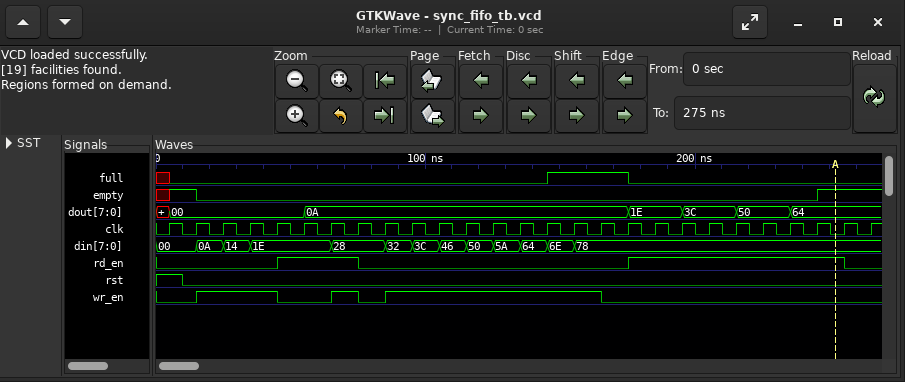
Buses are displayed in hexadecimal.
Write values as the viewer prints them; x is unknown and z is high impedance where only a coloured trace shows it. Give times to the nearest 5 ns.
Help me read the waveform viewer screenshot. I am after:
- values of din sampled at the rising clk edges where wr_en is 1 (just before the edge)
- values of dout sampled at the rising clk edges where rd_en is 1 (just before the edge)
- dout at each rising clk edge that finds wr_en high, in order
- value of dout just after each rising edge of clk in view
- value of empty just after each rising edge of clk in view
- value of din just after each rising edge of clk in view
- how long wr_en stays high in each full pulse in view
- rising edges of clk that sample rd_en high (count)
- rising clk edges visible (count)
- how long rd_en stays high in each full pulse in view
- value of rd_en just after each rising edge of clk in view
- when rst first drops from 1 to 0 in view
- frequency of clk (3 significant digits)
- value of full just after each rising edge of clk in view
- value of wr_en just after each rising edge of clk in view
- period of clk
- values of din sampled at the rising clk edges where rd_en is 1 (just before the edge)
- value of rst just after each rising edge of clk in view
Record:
0A, 14, 1E, 28, 32, 3C, 46, 50, 5A, 64, 6E, 78
00, 0A, 0A, 1E, 1E, 3C, 3C, 50, 50, 64, 64
00, 00, 00, 0A, 0A, 0A, 0A, 0A, 0A, 0A, 0A, 0A
00, 00, 00, 00, 00, 0A, 0A, 0A, 0A, 0A, 0A, 0A, 0A, 0A, 0A, 0A, 0A, 1E, 1E, 3C, 3C, 50, 50, 64, 64, 64, 64
1 0 0 0 0 0 0 0 0 0 0 0 0 0 0 0 0 0 0 0 0 0 0 0 1 1 1
00, 0A, 14, 1E, 1E, 1E, 28, 28, 32, 3C, 46, 50, 5A, 64, 6E, 78, 78, 78, 78, 78, 78, 78, 78, 78, 78, 78, 78
30 ns, 10 ns, 80 ns
11
27
30 ns, 80 ns
0 0 0 0 1 1 1 0 0 0 0 0 0 0 0 0 0 1 1 1 1 1 1 1 1 0 0
10 ns
100 MHz
0 0 0 0 0 0 0 0 0 0 0 0 0 0 1 1 1 0 0 0 0 0 0 0 0 0 0
0 1 1 1 0 0 1 0 1 1 1 1 1 1 1 1 0 0 0 0 0 0 0 0 0 0 0
10 ns
1E, 1E, 28, 78, 78, 78, 78, 78, 78, 78, 78
1 0 0 0 0 0 0 0 0 0 0 0 0 0 0 0 0 0 0 0 0 0 0 0 0 0 0
